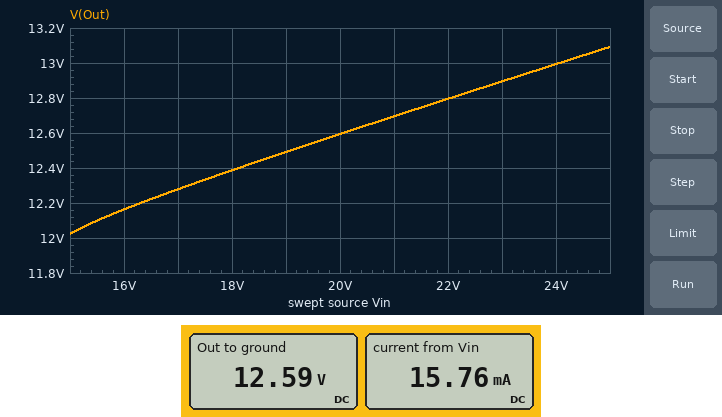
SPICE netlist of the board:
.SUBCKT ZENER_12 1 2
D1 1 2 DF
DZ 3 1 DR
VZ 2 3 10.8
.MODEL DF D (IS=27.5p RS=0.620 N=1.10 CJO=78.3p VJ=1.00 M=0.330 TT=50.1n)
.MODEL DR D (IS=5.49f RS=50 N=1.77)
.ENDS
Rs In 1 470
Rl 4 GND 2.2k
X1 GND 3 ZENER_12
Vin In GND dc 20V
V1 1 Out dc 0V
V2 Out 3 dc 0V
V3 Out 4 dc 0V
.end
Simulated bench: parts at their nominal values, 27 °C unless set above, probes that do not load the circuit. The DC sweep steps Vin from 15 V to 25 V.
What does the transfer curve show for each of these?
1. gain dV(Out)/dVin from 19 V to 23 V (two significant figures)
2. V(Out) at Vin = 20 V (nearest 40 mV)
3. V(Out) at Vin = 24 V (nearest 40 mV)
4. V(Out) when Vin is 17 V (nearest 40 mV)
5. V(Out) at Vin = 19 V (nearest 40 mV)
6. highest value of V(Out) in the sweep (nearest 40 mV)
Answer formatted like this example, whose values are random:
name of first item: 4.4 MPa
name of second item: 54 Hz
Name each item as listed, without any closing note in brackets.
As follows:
gain dV(Out)/dVin from 19 V to 23 V: 0.10 V/V
V(Out) at Vin = 20 V: 12.60 V
V(Out) at Vin = 24 V: 13.00 V
V(Out) when Vin is 17 V: 12.28 V
V(Out) at Vin = 19 V: 12.48 V
highest value of V(Out) in the sweep: 13.08 V
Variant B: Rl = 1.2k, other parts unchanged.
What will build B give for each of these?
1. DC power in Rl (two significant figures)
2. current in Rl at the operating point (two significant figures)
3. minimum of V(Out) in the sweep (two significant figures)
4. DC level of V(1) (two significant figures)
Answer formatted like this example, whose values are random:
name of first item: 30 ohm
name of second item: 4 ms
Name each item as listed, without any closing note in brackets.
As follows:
DC power in Rl: 130 mW
current in Rl at the operating point: 10 mA
minimum of V(Out) in the sweep: 11 V
DC level of V(1): 12 V
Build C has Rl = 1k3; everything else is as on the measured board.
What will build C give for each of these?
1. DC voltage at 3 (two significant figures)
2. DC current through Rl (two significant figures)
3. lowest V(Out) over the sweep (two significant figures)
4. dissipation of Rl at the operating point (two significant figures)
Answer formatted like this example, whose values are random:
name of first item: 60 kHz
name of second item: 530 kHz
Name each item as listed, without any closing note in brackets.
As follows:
DC voltage at 3: 12 V
DC current through Rl: 9.5 mA
lowest V(Out) over the sweep: 11 V
dissipation of Rl at the operating point: 120 mW
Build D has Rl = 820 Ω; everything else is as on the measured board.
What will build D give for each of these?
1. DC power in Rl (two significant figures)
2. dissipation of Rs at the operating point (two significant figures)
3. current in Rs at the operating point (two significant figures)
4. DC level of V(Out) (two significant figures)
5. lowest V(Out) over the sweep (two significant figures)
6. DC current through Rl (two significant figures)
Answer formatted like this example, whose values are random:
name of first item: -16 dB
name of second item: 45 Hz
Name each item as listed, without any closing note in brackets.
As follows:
DC power in Rl: 180 mW
dissipation of Rs at the operating point: 130 mW
current in Rs at the operating point: 17 mA
DC level of V(Out): 12 V
lowest V(Out) over the sweep: 9.5 V
DC current through Rl: 15 mA
